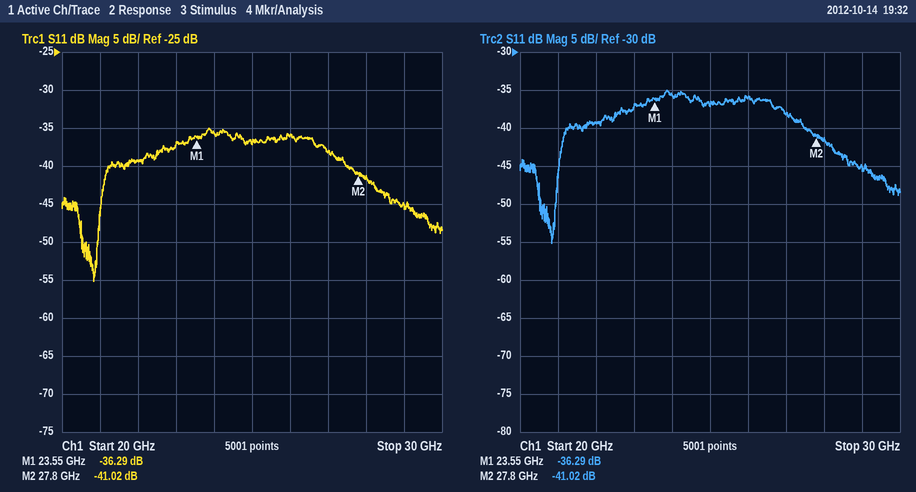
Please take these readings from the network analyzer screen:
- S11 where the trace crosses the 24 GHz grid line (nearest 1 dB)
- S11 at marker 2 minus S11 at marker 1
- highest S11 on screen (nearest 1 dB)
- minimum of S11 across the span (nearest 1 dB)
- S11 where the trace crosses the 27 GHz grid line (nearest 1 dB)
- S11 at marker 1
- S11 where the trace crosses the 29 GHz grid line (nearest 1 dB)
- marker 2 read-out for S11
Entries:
-36 dB
-4.73 dB
-35 dB
-55 dB
-38 dB
-36.29 dB
-45 dB
-41.02 dB
